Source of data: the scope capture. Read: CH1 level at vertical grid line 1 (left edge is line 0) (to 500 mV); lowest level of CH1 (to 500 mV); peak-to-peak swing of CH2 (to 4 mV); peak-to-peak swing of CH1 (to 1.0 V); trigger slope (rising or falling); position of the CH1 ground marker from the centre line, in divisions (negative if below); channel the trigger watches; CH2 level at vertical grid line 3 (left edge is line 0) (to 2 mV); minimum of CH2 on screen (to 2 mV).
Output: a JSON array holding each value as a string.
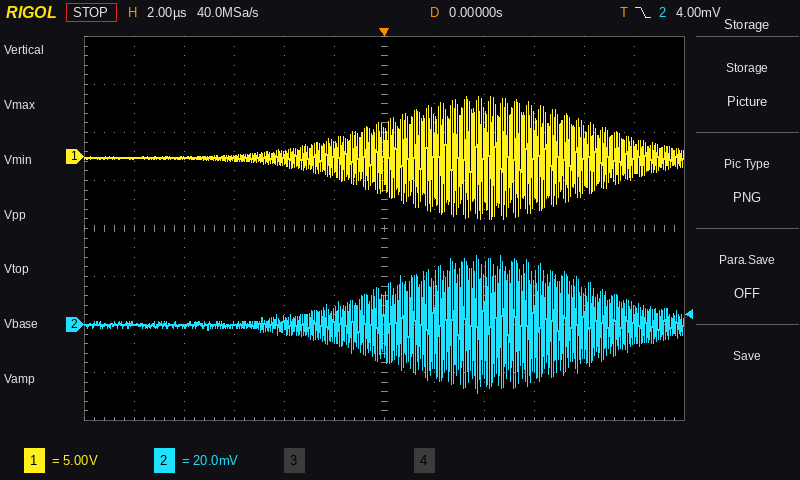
["0.0 V", "-6.5 V", "56 mV", "13.0 V", "falling", "+1.5 div", "CH2", "0 mV", "-28 mV"]
